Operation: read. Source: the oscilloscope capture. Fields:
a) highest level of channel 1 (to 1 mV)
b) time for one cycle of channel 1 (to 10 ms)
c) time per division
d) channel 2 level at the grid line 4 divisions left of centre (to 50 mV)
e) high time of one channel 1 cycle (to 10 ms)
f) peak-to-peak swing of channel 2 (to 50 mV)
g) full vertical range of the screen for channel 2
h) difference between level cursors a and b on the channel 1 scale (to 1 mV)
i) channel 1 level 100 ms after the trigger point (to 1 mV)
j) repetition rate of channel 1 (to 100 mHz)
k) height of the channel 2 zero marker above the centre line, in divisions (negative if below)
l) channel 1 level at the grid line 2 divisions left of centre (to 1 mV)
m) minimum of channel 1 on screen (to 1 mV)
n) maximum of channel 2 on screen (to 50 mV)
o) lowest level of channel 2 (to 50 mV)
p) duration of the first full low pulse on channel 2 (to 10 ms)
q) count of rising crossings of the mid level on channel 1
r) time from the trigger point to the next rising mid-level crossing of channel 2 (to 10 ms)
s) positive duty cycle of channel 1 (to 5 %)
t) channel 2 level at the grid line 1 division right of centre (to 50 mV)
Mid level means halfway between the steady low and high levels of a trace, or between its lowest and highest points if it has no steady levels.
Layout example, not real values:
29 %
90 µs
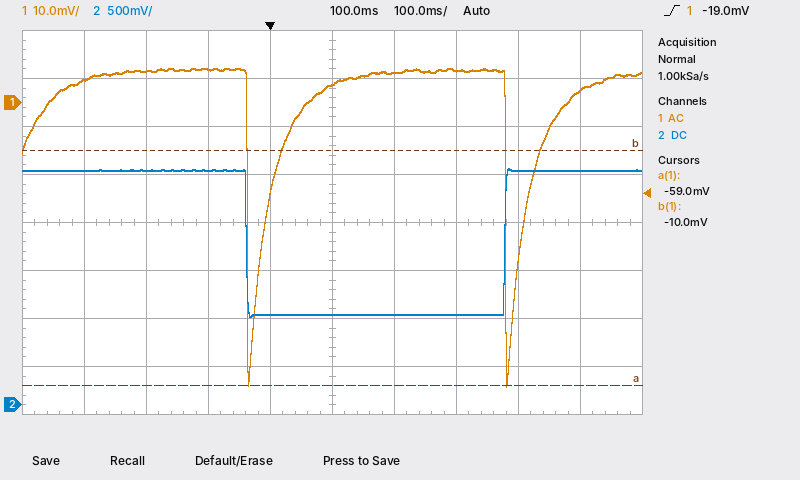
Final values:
7 mV
420 ms
100 ms
2.45 V
390 ms
1.55 V
4 V
49 mV
4 mV
2.4 Hz
-3.8 div
7 mV
-59 mV
2.45 V
900 mV
420 ms
2
380 ms
95 %
950 mV
